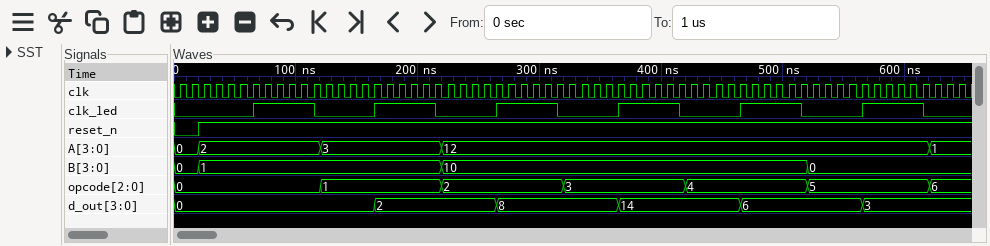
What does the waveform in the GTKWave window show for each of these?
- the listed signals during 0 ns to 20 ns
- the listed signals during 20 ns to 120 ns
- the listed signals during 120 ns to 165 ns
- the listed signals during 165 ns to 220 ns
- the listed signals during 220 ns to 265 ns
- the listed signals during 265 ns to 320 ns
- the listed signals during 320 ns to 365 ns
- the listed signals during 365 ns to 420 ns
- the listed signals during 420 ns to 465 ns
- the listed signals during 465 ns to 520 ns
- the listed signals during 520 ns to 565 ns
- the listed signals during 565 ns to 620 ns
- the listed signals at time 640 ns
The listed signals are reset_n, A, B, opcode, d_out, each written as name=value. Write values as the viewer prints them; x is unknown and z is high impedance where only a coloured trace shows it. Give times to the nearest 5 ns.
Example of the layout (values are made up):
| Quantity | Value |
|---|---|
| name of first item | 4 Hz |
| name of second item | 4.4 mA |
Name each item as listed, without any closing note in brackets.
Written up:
| Quantity | Value |
|---|---|
| the listed signals during 0 ns to 20 ns | reset_n=0, A=0, B=0, opcode=0, d_out=0 |
| the listed signals during 20 ns to 120 ns | reset_n=1, A=2, B=1, opcode=0, d_out=0 |
| the listed signals during 120 ns to 165 ns | reset_n=1, A=3, B=1, opcode=1, d_out=0 |
| the listed signals during 165 ns to 220 ns | reset_n=1, A=3, B=1, opcode=1, d_out=2 |
| the listed signals during 220 ns to 265 ns | reset_n=1, A=12, B=10, opcode=2, d_out=2 |
| the listed signals during 265 ns to 320 ns | reset_n=1, A=12, B=10, opcode=2, d_out=8 |
| the listed signals during 320 ns to 365 ns | reset_n=1, A=12, B=10, opcode=3, d_out=8 |
| the listed signals during 365 ns to 420 ns | reset_n=1, A=12, B=10, opcode=3, d_out=14 |
| the listed signals during 420 ns to 465 ns | reset_n=1, A=12, B=10, opcode=4, d_out=14 |
| the listed signals during 465 ns to 520 ns | reset_n=1, A=12, B=10, opcode=4, d_out=6 |
| the listed signals during 520 ns to 565 ns | reset_n=1, A=12, B=0, opcode=5, d_out=6 |
| the listed signals during 565 ns to 620 ns | reset_n=1, A=12, B=0, opcode=5, d_out=3 |
| the listed signals at time 640 ns | reset_n=1, A=1, B=0, opcode=6, d_out=3 |
